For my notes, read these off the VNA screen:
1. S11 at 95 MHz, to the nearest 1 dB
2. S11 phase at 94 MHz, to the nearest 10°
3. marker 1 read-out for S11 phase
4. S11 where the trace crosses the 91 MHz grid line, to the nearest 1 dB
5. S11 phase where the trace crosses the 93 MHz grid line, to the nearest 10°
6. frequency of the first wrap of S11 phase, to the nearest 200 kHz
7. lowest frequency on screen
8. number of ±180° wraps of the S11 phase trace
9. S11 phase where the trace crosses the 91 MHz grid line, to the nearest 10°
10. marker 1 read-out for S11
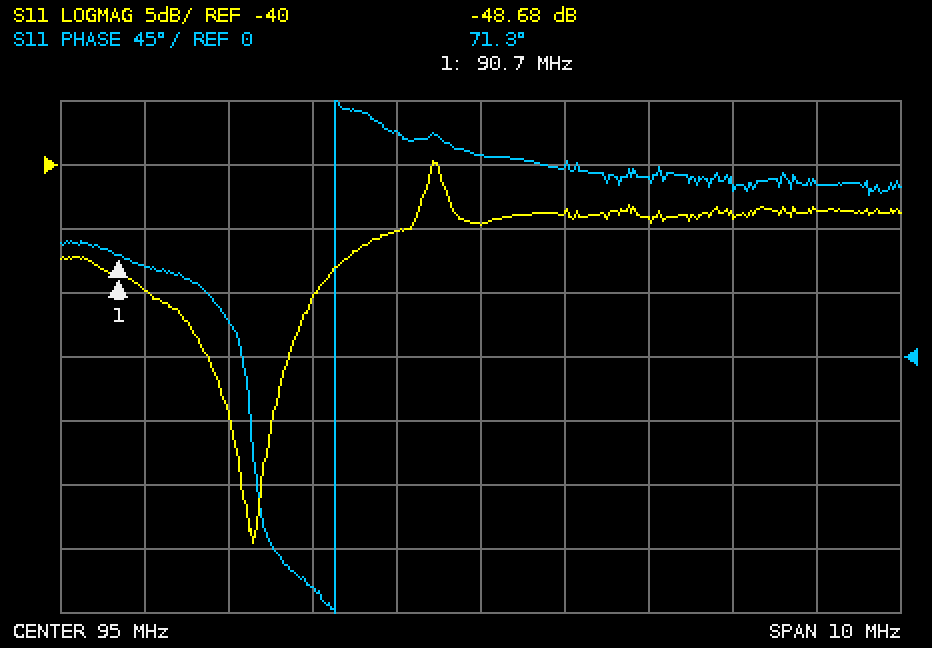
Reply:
-45 dB
160°
71.3°
-50 dB
-160°
93.2 MHz
90 MHz
1
60°
-48.68 dB
